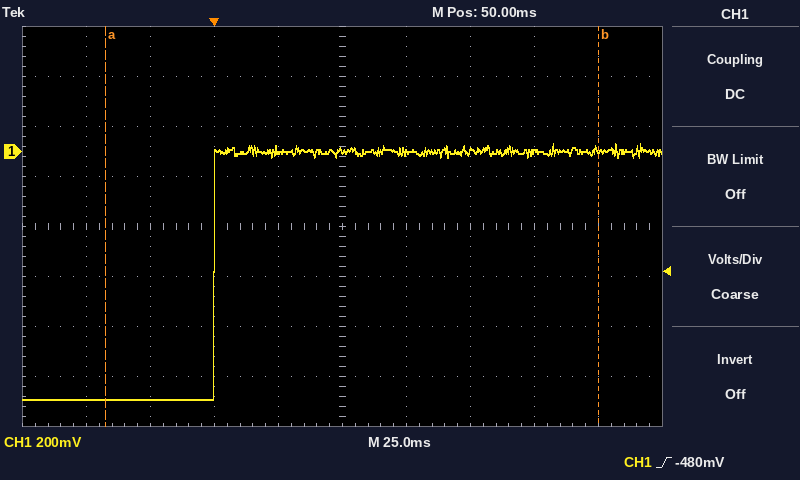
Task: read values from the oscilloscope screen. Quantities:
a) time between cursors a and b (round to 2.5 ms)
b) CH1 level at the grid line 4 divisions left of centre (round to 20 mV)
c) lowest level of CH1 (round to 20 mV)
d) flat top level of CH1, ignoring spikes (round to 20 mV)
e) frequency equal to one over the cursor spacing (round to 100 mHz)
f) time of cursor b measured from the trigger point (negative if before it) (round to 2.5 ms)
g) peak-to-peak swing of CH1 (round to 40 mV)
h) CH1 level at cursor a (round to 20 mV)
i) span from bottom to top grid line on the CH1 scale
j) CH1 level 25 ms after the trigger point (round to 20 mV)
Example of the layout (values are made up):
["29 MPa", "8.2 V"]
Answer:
["192.5 ms", "-1.00 V", "-1.00 V", "0 mV", "5.2 Hz", "+150.0 ms", "1.04 V", "-1.00 V", "1.6 V", "0 mV"]
